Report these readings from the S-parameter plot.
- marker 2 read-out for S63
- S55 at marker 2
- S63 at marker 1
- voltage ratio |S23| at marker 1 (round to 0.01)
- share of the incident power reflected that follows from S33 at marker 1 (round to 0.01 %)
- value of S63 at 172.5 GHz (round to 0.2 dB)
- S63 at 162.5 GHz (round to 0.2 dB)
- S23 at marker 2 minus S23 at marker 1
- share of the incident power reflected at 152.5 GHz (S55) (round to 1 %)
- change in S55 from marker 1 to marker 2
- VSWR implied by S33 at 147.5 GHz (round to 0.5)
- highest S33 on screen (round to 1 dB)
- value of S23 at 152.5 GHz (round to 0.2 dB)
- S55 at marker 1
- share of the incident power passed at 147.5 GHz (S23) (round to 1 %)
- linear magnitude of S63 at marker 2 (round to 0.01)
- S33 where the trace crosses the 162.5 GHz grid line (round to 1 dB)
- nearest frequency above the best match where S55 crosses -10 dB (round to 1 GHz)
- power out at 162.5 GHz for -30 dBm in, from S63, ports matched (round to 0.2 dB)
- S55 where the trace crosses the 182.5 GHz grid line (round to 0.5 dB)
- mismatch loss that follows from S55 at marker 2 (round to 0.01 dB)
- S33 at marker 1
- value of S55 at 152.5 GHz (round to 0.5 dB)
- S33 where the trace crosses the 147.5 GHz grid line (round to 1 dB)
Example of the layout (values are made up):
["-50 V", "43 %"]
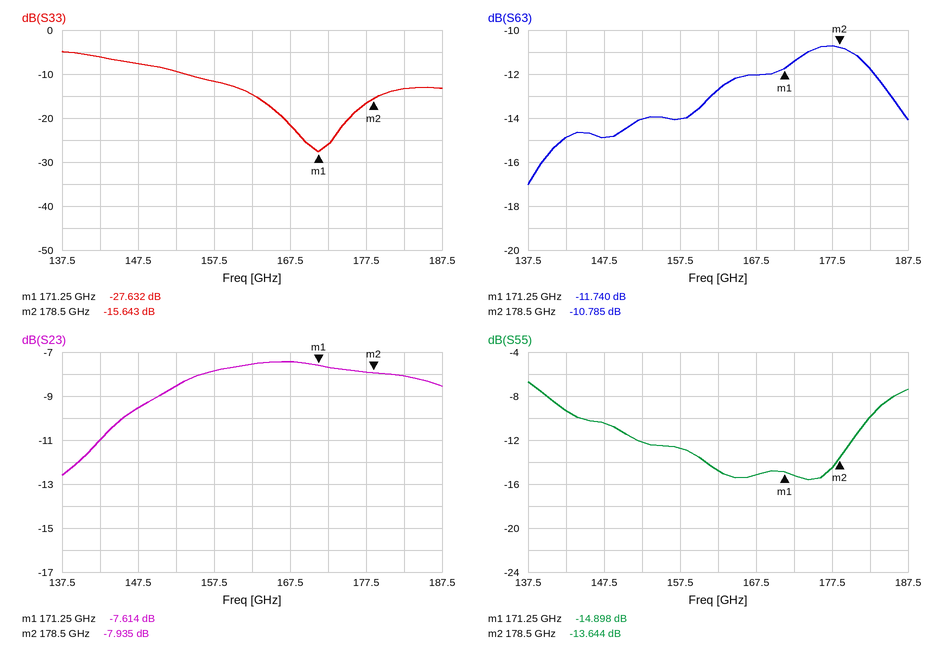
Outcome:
["-10.785 dB", "-13.644 dB", "-11.740 dB", "0.42", "0.17 %", "-11.4 dB", "-12.8 dB", "-0.321 dB", "6 %", "1.254 dB", "2.5", "-5 dB", "-8.6 dB", "-14.898 dB", "11 %", "0.29", "-15 dB", "182 GHz", "-42.8 dBm", "-10.0 dB", "0.19 dB", "-27.632 dB", "-12.0 dB", "-8 dB"]
